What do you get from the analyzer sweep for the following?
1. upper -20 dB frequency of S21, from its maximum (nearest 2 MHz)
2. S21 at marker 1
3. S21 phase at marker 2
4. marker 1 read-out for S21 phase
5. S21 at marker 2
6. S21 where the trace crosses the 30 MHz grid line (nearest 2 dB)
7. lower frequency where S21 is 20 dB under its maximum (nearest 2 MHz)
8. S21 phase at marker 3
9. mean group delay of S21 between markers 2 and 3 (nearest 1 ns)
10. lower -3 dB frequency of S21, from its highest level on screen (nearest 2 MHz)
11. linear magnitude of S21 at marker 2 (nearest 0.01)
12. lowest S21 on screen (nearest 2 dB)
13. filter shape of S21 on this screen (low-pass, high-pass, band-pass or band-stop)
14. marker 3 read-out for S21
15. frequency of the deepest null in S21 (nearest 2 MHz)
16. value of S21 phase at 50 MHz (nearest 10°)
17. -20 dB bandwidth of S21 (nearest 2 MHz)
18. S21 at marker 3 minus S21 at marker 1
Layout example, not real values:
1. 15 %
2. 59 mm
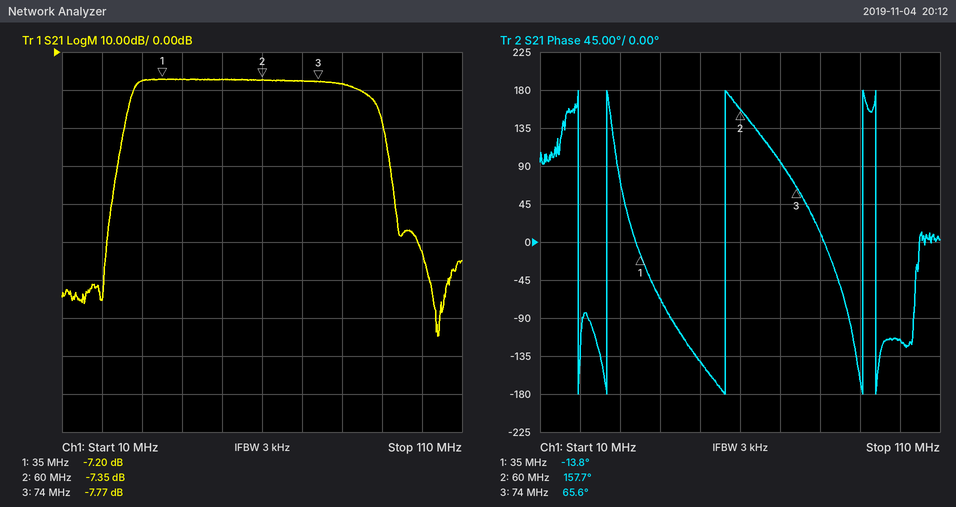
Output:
1. 92 MHz
2. -7.20 dB
3. 157.7°
4. -13.8°
5. -7.35 dB
6. -8 dB
7. 24 MHz
8. 65.6°
9. 18 ns
10. 28 MHz
11. 0.43
12. -74 dB
13. band-pass
14. -7.77 dB
15. 104 MHz
16. -140°
17. 68 MHz
18. -0.57 dB
